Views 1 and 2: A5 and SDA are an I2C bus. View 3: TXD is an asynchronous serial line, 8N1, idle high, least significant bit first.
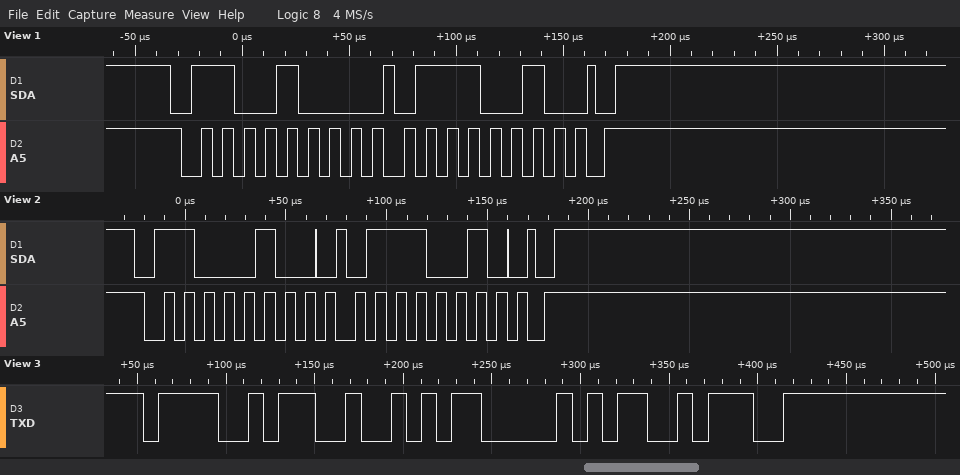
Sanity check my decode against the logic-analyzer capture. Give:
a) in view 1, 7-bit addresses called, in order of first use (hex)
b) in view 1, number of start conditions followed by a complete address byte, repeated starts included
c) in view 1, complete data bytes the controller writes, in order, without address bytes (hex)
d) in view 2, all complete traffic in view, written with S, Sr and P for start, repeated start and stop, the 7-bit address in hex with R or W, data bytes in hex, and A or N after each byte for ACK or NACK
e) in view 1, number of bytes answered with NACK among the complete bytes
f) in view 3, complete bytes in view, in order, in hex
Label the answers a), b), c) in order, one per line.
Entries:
a) 0x64
b) 1
c) 72
d) S 62W A 72 A P
e) 0
f) 4F 52 50 3A
